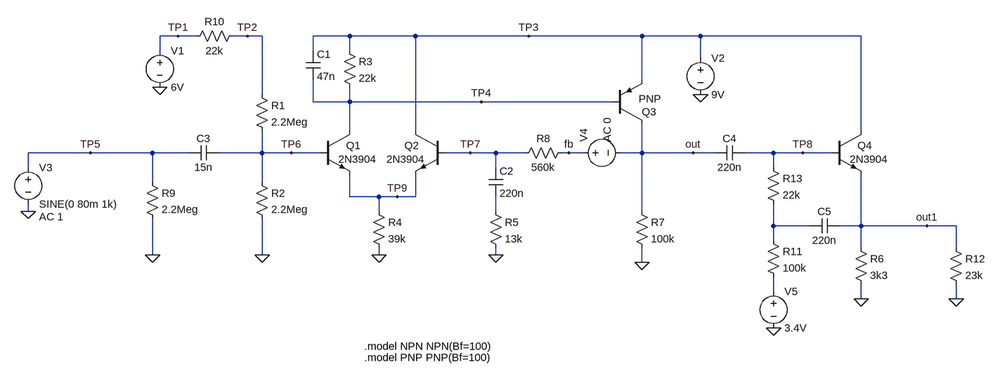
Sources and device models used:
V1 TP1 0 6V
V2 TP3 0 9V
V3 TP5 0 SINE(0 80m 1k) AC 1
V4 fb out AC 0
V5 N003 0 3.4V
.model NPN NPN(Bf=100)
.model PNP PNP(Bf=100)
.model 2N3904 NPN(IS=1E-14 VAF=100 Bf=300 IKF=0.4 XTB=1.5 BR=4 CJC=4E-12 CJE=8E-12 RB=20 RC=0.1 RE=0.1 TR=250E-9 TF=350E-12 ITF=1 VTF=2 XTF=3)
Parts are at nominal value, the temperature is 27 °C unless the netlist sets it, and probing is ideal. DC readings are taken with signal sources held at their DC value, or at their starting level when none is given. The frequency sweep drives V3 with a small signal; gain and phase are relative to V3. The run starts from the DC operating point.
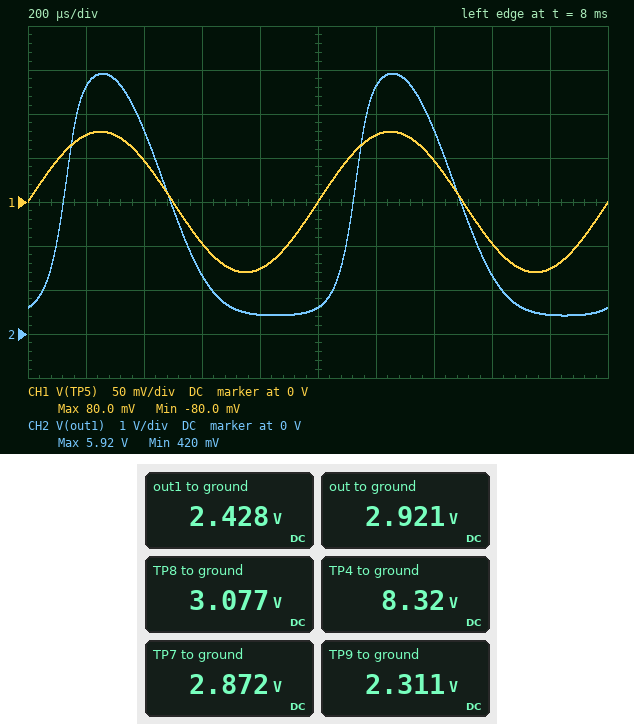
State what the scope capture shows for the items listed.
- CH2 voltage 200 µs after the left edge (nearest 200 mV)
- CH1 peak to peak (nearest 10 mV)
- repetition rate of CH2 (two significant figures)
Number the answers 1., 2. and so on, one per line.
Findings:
1. 5.6 V
2. 160 mV
3. 1.0 kHz
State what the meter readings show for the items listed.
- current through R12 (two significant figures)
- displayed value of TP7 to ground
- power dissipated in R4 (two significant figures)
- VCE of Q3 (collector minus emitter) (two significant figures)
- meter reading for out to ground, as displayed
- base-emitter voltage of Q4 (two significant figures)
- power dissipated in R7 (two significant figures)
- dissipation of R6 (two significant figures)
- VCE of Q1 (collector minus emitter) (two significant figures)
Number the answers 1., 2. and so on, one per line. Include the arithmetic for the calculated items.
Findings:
1. (2.428 V) / 23 kΩ = 110 µA
2. 2.872 V
3. (2.311 V)^2 / 39 kΩ = 140 µW
4. 2.921 V - 9 V = -6.1 V
5. 2.921 V
6. 3.077 V - 2.428 V = 650 mV
7. (2.921 V)^2 / 100 kΩ = 85 µW
8. (2.428 V)^2 / 3.3 kΩ = 1.8 mW
9. 8.32 V - 2.311 V = 6.0 V
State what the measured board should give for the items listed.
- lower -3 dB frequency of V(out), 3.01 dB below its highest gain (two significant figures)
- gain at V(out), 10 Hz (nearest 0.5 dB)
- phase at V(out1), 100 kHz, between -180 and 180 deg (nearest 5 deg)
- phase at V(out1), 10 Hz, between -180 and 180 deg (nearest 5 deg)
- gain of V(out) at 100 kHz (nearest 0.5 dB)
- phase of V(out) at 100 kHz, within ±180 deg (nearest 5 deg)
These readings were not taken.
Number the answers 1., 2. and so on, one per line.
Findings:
1. 55 Hz
2. 15.0 dB
3. -95 deg
4. 150 deg
5. 4.0 dB
6. -95 deg
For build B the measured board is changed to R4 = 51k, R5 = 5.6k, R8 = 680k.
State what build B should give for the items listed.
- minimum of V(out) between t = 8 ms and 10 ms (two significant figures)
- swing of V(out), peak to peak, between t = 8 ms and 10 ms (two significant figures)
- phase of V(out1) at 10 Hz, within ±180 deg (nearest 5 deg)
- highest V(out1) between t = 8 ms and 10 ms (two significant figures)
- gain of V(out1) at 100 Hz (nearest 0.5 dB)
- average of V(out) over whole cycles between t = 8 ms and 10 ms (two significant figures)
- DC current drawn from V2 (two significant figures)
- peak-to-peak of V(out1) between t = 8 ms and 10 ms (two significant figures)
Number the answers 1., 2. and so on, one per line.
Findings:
1. 780 mV
2. 8.1 V
3. 155 deg
4. 8.4 V
5. 37.0 dB
6. 2.9 V
7. 910 µA
8. 8.0 V
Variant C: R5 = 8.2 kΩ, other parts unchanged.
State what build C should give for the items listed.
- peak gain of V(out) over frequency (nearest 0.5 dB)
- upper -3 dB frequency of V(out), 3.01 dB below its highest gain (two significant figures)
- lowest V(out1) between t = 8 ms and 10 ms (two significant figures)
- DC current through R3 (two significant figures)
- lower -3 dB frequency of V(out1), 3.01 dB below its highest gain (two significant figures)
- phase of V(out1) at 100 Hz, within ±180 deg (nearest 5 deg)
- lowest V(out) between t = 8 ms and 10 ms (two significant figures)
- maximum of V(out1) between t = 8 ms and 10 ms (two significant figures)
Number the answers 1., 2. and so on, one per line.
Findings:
1. 36.0 dB
2. 2.6 kHz
3. 360 mV
4. 31 µA
5. 78 Hz
6. 45 deg
7. 800 mV
8. 7.8 V
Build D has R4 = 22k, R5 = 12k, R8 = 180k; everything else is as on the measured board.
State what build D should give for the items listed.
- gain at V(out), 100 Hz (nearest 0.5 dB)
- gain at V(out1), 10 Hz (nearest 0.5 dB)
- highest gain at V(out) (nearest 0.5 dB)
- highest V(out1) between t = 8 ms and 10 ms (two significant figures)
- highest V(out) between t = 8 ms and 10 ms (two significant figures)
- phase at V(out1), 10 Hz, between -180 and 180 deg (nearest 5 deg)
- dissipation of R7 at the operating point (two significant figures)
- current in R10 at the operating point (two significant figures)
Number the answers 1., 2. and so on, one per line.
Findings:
1. 22.5 dB
2. 5.5 dB
3. 24.0 dB
4. 3.7 V
5. 4.2 V
6. 140 deg
7. 86 µW
8. 1.4 µA
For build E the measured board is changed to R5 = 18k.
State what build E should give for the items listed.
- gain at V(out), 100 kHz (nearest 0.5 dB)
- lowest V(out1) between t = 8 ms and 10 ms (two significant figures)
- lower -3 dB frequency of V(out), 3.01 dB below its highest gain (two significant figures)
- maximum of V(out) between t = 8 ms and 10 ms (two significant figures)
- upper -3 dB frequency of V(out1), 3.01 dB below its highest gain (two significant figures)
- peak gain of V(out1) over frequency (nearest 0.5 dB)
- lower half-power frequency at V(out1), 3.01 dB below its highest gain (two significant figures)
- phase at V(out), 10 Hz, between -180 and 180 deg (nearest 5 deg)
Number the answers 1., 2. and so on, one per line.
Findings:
1. 4.0 dB
2. 530 mV
3. 42 Hz
4. 5.5 V
5. 5.2 kHz
6. 30.0 dB
7. 37 Hz
8. 110 deg
